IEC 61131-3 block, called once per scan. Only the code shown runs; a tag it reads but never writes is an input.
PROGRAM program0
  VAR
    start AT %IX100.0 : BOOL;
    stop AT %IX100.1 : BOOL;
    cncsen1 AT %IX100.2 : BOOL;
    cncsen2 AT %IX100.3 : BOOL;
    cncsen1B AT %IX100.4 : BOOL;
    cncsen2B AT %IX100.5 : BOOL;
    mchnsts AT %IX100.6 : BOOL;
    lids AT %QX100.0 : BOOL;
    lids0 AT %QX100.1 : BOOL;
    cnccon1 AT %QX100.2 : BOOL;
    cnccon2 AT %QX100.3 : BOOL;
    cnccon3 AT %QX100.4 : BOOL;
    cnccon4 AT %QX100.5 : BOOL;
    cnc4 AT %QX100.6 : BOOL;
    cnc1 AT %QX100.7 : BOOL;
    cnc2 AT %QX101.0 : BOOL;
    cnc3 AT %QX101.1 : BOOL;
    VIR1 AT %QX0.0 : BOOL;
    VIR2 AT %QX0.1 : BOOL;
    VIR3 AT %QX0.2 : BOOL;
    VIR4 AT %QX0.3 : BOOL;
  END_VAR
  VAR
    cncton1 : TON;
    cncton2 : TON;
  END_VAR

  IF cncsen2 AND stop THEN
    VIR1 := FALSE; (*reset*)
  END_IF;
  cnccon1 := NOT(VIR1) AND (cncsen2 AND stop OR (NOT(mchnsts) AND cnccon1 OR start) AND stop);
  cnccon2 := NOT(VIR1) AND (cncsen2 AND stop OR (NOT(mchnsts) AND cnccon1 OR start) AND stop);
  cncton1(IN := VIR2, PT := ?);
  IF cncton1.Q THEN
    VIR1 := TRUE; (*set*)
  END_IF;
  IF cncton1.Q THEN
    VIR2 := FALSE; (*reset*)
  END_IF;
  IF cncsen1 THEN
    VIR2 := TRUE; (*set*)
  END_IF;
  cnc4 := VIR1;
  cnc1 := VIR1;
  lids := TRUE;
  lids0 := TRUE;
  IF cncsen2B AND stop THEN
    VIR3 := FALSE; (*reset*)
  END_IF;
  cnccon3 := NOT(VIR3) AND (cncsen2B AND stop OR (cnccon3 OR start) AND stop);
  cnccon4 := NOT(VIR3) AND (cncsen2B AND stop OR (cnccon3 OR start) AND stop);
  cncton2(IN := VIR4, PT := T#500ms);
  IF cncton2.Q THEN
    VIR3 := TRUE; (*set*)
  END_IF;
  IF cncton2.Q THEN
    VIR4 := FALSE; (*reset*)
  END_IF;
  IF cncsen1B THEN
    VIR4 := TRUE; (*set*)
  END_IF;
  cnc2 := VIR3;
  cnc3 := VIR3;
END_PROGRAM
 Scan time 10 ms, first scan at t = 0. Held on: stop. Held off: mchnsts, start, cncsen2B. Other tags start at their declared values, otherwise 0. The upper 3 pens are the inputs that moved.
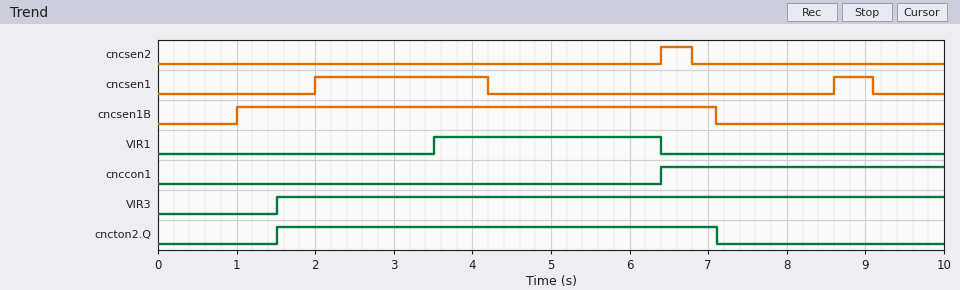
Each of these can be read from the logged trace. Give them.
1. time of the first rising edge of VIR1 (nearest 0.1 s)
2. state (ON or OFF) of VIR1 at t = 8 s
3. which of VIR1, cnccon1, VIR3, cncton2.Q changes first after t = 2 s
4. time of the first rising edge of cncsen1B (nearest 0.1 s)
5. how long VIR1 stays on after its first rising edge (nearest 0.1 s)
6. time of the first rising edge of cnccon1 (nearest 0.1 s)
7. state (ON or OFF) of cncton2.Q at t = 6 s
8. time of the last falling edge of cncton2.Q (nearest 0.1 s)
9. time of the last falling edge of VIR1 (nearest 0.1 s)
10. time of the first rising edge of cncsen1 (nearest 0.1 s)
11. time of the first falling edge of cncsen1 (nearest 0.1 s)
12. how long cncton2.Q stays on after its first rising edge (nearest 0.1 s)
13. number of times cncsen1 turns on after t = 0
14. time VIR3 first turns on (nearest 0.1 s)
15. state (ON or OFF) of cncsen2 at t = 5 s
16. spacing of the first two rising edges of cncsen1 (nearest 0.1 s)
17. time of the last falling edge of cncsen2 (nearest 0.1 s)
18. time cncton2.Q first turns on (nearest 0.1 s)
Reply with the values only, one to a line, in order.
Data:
3.5 s
OFF
VIR1
1.0 s
2.9 s
6.4 s
ON
7.1 s
6.4 s
2.0 s
4.2 s
5.6 s
2
1.5 s
OFF
6.6 s
6.8 s
1.5 s
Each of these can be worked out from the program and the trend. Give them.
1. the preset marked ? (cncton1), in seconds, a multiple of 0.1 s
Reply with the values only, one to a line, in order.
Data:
1.5 s
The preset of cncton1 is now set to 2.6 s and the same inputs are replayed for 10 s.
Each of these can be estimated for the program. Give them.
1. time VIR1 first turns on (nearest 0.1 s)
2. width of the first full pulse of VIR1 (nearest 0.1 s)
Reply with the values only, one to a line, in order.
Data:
4.6 s
1.8 s
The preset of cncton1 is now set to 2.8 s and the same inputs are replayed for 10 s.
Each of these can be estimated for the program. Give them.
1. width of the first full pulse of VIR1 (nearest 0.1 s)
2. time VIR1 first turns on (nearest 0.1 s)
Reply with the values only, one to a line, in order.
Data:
1.6 s
4.8 s
